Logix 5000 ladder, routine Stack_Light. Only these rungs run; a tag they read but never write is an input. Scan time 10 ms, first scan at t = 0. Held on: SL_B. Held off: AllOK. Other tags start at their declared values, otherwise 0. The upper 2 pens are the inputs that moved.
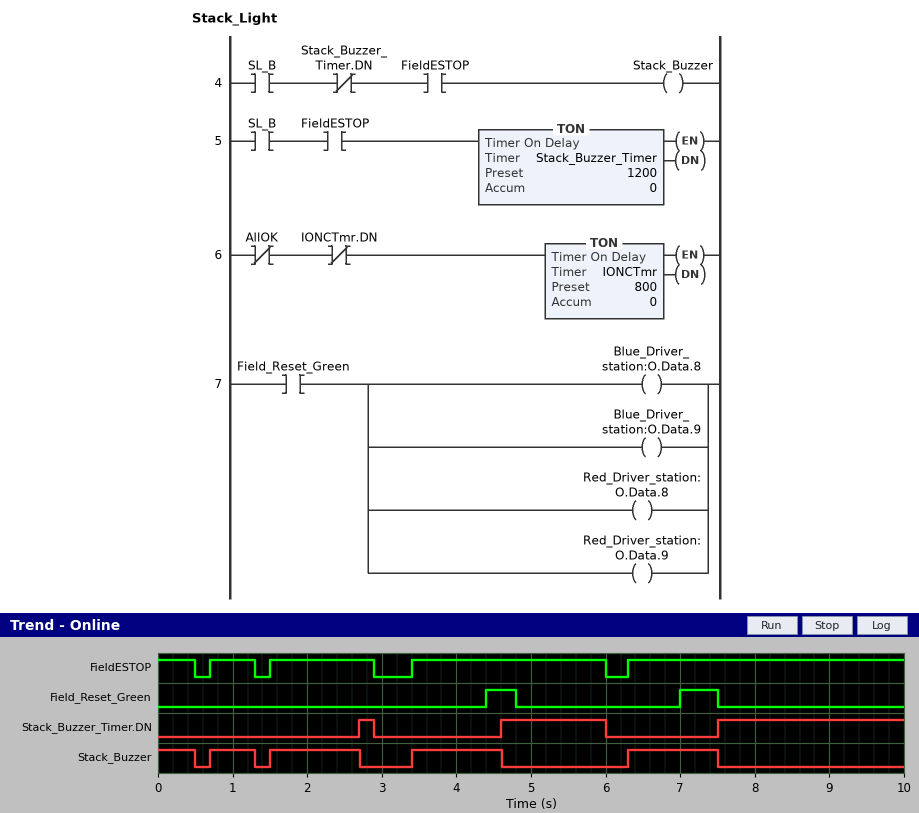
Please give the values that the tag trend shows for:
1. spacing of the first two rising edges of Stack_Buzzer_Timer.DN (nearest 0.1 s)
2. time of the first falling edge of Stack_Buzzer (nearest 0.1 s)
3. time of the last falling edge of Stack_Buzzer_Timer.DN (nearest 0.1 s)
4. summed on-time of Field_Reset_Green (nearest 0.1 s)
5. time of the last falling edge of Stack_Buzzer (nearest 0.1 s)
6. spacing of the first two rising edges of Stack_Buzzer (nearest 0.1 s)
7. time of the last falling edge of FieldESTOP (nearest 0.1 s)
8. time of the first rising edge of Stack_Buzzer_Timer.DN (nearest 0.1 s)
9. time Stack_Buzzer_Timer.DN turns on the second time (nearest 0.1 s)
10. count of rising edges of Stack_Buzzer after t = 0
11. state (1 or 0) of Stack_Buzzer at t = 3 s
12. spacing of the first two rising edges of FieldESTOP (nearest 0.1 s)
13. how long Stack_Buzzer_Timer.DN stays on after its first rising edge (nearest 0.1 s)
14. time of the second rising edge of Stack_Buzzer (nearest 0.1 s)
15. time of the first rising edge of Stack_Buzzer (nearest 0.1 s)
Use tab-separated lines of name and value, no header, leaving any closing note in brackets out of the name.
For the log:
spacing of the first two rising edges of Stack_Buzzer_Timer.DN	1.9 s
time of the first falling edge of Stack_Buzzer	0.5 s
time of the last falling edge of Stack_Buzzer_Timer.DN	6.0 s
summed on-time of Field_Reset_Green	0.9 s
time of the last falling edge of Stack_Buzzer	7.5 s
spacing of the first two rising edges of Stack_Buzzer	0.8 s
time of the last falling edge of FieldESTOP	6.0 s
time of the first rising edge of Stack_Buzzer_Timer.DN	2.7 s
time Stack_Buzzer_Timer.DN turns on the second time	4.6 s
count of rising edges of Stack_Buzzer after t = 0	4
state (1 or 0) of Stack_Buzzer at t = 3 s	0
spacing of the first two rising edges of FieldESTOP	0.8 s
how long Stack_Buzzer_Timer.DN stays on after its first rising edge	0.2 s
time of the second rising edge of Stack_Buzzer	1.5 s
time of the first rising edge of Stack_Buzzer	0.7 s
